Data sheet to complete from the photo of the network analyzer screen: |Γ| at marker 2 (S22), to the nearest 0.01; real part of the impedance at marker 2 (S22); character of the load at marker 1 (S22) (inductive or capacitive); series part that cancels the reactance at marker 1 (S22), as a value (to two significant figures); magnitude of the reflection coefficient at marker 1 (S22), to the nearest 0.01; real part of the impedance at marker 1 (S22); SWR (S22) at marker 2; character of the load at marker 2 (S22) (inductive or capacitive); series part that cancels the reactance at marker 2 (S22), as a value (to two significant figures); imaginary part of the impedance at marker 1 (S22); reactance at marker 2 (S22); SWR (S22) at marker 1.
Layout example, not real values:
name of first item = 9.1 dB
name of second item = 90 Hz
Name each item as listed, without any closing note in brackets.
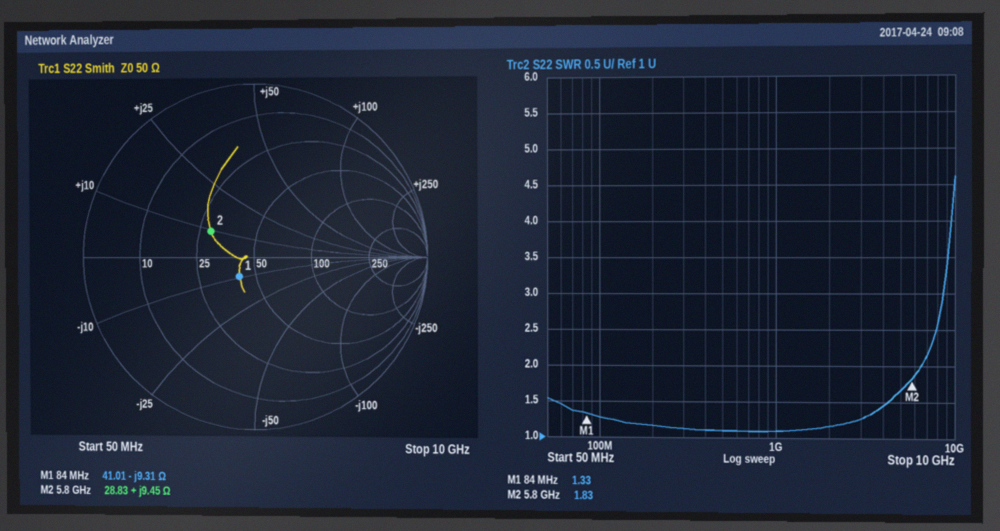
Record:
|Γ| at marker 2 (S22), to the nearest 0.01 = 0.29
real part of the impedance at marker 2 = 28.83 Ω
character of the load at marker 1 (S22) = capacitive
series part that cancels the reactance at marker 1 (S22), as a value = 18 nH
magnitude of the reflection coefficient at marker 1 (S22), to the nearest 0.01 = 0.14
real part of the impedance at marker 1 = 41.01 Ω
SWR (S22) at marker 2 = 1.83
character of the load at marker 2 (S22) = inductive
series part that cancels the reactance at marker 2 (S22), as a value = 2.9 pF
imaginary part of the impedance at marker 1 = -9.31 Ω
reactance at marker 2 = +9.45 Ω
SWR (S22) at marker 1 = 1.33
